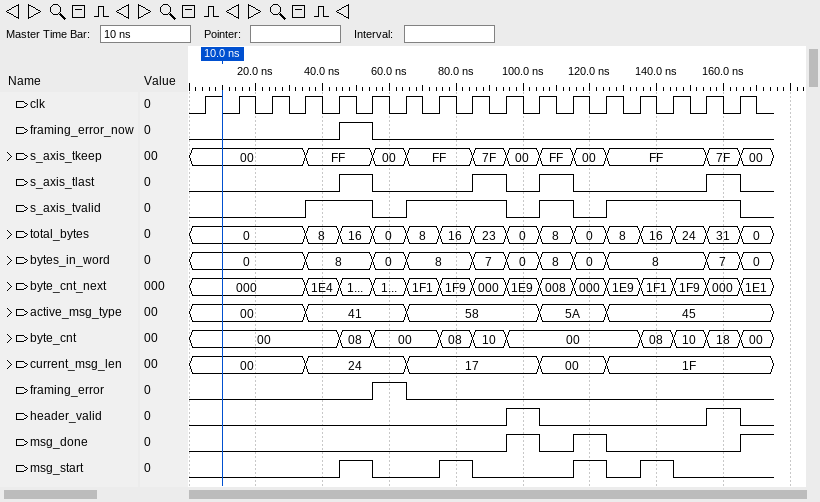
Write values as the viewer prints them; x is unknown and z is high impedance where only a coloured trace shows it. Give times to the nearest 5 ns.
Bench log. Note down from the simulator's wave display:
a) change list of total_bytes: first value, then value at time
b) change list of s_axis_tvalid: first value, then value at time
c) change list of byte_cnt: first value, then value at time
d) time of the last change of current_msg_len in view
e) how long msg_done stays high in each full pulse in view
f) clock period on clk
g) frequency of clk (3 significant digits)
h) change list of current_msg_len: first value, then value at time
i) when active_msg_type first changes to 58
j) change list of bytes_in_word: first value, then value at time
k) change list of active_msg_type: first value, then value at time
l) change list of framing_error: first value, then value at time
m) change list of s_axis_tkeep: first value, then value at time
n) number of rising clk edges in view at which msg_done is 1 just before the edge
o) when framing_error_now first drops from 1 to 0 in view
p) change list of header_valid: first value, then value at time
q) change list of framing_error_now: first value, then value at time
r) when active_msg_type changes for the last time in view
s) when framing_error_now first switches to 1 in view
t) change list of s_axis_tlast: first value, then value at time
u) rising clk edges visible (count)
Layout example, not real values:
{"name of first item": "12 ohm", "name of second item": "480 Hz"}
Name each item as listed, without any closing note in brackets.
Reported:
{"change list of total_bytes: first value, then value at time": "0, 8 at 35 ns, 16 at 45 ns, 0 at 55 ns, 8 at 65 ns, 16 at 75 ns, 23 at 85 ns, 0 at 95 ns, 8 at 105 ns, 0 at 115 ns, 8 at 125 ns, 16 at 135 ns, 24 at 145 ns, 31 at 155 ns, 0 at 165 ns", "change list of s_axis_tvalid: first value, then value at time": "0, 1 at 35 ns, 0 at 55 ns, 1 at 65 ns, 0 at 95 ns, 1 at 105 ns, 0 at 115 ns, 1 at 125 ns, 0 at 165 ns", "change list of byte_cnt: first value, then value at time": "00, 08 at 45 ns, 00 at 55 ns, 08 at 75 ns, 10 at 85 ns, 00 at 95 ns, 08 at 135 ns, 10 at 145 ns, 18 at 155 ns, 00 at 165 ns", "time of the last change of current_msg_len in view": "125 ns", "how long msg_done stays high in each full pulse in view": "10 ns, 10 ns", "clock period on clk": "10 ns", "frequency of clk": "100 MHz", "change list of current_msg_len: first value, then value at time": "00, 24 at 35 ns, 17 at 65 ns, 00 at 105 ns, 1F at 125 ns", "when active_msg_type first changes to 58": "65 ns", "change list of bytes_in_word: first value, then value at time": "0, 8 at 35 ns, 0 at 55 ns, 8 at 65 ns, 7 at 85 ns, 0 at 95 ns, 8 at 105 ns, 0 at 115 ns, 8 at 125 ns, 7 at 155 ns, 0 at 165 ns", "change list of active_msg_type: first value, then value at time": "00, 41 at 35 ns, 58 at 65 ns, 5A at 105 ns, 45 at 125 ns", "change list of framing_error: first value, then value at time": "0, 1 at 55 ns, 0 at 65 ns", "change list of s_axis_tkeep: first value, then value at time": "00, FF at 35 ns, 00 at 55 ns, FF at 65 ns, 7F at 85 ns, 00 at 95 ns, FF at 105 ns, 00 at 115 ns, FF at 125 ns, 7F at 155 ns, 00 at 165 ns", "number of rising clk edges in view at which msg_done is 1 just before the edge": "2", "when framing_error_now first drops from 1 to 0 in view": "55 ns", "change list of header_valid: first value, then value at time": "0, 1 at 95 ns, 0 at 105 ns, 1 at 155 ns, 0 at 165 ns", "change list of framing_error_now: first value, then value at time": "0, 1 at 45 ns, 0 at 55 ns", "when active_msg_type changes for the last time in view": "125 ns", "when framing_error_now first switches to 1 in view": "45 ns", "change list of s_axis_tlast: first value, then value at time": "0, 1 at 45 ns, 0 at 55 ns, 1 at 85 ns, 0 at 95 ns, 1 at 105 ns, 0 at 115 ns, 1 at 155 ns, 0 at 165 ns", "rising clk edges visible": "17"}
